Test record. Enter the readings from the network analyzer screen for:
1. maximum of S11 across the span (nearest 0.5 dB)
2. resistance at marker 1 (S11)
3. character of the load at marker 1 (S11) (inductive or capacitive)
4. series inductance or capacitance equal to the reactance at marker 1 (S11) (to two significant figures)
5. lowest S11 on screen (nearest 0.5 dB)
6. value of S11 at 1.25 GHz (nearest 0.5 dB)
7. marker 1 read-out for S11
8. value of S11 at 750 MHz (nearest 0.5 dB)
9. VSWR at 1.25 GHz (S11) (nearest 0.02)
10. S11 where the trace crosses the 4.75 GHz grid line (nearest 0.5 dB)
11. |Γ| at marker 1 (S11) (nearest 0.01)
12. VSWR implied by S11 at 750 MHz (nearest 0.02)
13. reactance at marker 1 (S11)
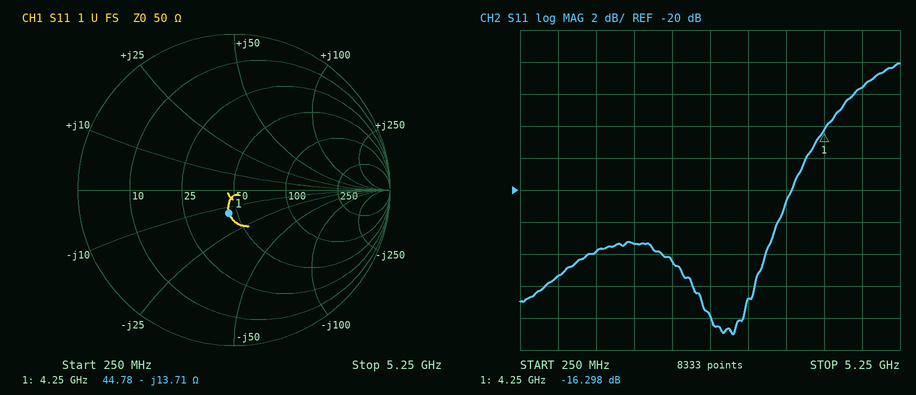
-12.0 dB
44.78 Ω
capacitive
2.7 pF
-29.0 dB
-24.0 dB
-16.298 dB
-25.5 dB
1.14
-13.5 dB
0.15
1.12
-13.71 Ω
